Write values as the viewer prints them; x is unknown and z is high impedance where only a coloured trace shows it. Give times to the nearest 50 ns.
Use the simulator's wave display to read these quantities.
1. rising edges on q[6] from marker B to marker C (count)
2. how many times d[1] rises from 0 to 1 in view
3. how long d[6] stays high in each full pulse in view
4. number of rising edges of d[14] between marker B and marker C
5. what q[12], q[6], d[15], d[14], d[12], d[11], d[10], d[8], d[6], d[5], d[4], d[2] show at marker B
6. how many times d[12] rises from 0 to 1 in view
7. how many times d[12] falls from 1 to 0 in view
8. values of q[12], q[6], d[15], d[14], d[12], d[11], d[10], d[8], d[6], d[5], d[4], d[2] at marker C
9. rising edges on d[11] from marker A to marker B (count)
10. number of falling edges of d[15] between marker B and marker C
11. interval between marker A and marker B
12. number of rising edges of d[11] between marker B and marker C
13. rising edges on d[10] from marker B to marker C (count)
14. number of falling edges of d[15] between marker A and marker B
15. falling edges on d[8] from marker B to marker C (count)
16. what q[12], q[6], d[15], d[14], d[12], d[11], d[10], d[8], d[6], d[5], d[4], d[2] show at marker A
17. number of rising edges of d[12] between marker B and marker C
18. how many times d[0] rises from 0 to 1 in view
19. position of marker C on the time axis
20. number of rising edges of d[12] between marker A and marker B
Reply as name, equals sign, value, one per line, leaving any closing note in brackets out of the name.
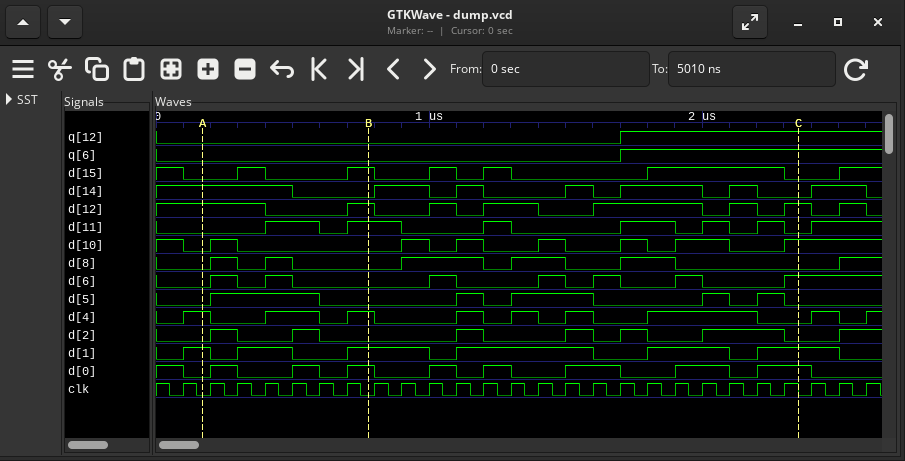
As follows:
rising edges on q[6] from marker B to marker C = 1
how many times d[1] rises from 0 to 1 in view = 6
how long d[6] stays high in each full pulse in view = 100 ns, 100 ns, 100 ns, 100 ns, 100 ns, 100 ns
number of rising edges of d[14] between marker B and marker C = 5
what q[12], q[6], d[15], d[14], d[12], d[11], d[10], d[8], d[6], d[5], d[4], d[2] show at marker B = q[12]=0, q[6]=0, d[15]=1, d[14]=0, d[12]=1, d[11]=1, d[10]=0, d[8]=0, d[6]=0, d[5]=0, d[4]=1, d[2]=0
how many times d[12] rises from 0 to 1 in view = 7
how many times d[12] falls from 1 to 0 in view = 8
values of q[12], q[6], d[15], d[14], d[12], d[11], d[10], d[8], d[6], d[5], d[4], d[2] at marker C = q[12]=1, q[6]=1, d[15]=0, d[14]=0, d[12]=1, d[11]=0, d[10]=1, d[8]=0, d[6]=1, d[5]=0, d[4]=0, d[2]=0
rising edges on d[11] from marker A to marker B = 2
number of falling edges of d[15] between marker B and marker C = 4
interval between marker A and marker B = 600 ns
number of rising edges of d[11] between marker B and marker C = 4
rising edges on d[10] from marker B to marker C = 6
number of falling edges of d[15] between marker A and marker B = 1
falling edges on d[8] from marker B to marker C = 3
what q[12], q[6], d[15], d[14], d[12], d[11], d[10], d[8], d[6], d[5], d[4], d[2] show at marker A = q[12]=0, q[6]=0, d[15]=0, d[14]=1, d[12]=1, d[11]=0, d[10]=0, d[8]=0, d[6]=0, d[5]=0, d[4]=1, d[2]=0
number of rising edges of d[12] between marker B and marker C = 5
how many times d[0] rises from 0 to 1 in view = 8
position of marker C on the time axis = 2350 ns
number of rising edges of d[12] between marker A and marker B = 1
